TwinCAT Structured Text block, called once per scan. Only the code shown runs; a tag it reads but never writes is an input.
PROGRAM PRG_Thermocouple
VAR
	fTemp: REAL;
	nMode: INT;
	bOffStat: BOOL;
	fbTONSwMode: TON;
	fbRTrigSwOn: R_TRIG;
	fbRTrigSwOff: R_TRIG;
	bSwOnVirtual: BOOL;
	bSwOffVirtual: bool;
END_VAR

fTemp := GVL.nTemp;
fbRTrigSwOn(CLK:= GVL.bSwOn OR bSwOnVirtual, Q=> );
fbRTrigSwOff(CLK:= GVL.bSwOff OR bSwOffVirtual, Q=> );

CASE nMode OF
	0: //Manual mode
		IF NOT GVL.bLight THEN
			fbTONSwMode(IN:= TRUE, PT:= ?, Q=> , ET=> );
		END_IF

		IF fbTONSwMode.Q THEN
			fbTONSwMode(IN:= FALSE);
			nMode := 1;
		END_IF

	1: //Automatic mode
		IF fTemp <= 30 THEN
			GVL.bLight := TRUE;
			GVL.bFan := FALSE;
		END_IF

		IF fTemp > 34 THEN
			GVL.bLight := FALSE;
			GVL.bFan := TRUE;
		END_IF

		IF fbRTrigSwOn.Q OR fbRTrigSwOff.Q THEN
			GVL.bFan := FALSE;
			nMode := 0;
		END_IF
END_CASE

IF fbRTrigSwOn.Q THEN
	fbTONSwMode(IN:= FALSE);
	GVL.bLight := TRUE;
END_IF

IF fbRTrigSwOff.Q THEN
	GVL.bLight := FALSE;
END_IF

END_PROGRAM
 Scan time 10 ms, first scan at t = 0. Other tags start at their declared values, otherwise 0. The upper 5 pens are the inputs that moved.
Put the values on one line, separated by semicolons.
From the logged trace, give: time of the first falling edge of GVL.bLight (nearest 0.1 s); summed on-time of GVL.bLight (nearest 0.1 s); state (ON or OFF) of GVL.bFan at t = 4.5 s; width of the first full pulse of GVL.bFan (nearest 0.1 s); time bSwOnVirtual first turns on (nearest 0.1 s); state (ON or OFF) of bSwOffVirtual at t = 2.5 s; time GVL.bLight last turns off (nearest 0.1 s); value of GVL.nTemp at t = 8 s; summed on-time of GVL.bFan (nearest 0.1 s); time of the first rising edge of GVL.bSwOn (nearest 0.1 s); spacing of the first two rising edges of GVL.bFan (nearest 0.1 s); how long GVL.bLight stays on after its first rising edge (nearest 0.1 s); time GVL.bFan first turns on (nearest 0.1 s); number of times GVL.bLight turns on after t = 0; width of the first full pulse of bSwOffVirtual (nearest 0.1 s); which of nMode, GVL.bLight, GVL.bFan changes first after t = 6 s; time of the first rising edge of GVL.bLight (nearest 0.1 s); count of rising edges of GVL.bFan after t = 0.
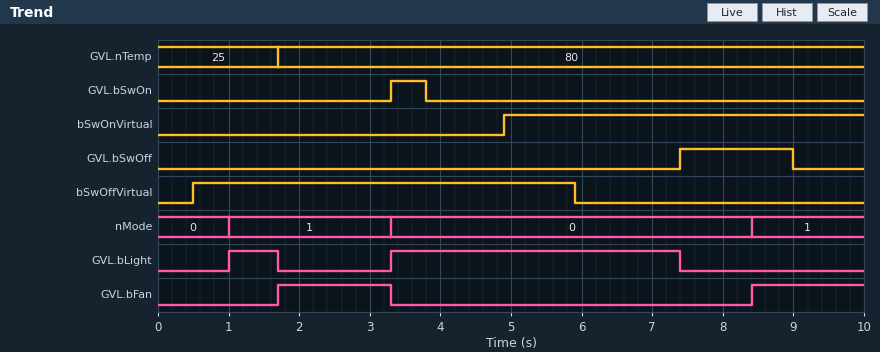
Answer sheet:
1.7 s; 4.8 s; OFF; 1.6 s; 4.9 s; ON; 7.4 s; 80; 3.2 s; 3.3 s; 6.7 s; 0.7 s; 1.7 s; 2; 5.4 s; GVL.bLight; 1.0 s; 2
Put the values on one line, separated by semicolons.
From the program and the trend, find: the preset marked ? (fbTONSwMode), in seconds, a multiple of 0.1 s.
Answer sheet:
1.0 s
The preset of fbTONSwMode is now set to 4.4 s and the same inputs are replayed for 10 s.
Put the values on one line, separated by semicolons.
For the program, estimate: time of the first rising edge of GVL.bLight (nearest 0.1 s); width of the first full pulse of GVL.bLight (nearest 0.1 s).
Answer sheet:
3.3 s; 4.1 s
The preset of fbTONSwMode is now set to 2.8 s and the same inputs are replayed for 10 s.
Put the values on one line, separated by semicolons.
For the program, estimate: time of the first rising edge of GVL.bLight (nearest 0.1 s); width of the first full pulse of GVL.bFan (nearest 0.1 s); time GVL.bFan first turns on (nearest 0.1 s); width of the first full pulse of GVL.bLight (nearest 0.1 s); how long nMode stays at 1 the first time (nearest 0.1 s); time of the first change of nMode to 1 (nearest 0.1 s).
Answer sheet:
3.3 s; 0.5 s; 2.8 s; 4.1 s; 0.5 s; 2.8 s
